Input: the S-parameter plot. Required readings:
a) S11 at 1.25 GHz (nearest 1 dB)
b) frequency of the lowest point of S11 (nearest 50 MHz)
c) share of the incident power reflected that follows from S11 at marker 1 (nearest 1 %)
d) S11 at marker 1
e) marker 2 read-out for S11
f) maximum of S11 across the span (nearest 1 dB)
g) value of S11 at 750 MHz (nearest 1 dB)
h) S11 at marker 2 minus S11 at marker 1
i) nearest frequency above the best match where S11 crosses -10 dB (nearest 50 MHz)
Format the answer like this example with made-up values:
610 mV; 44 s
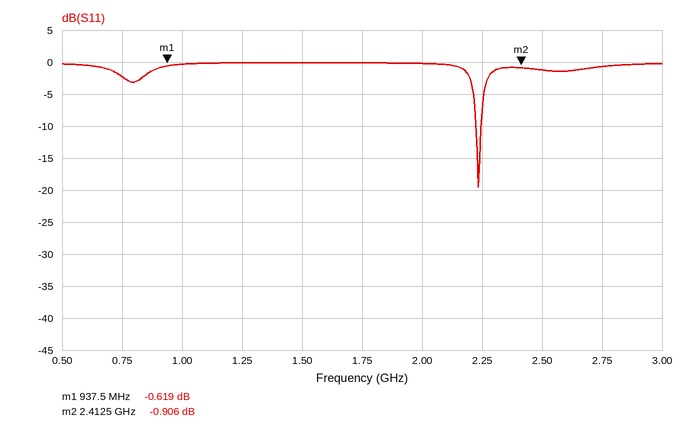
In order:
0 dB; 2.25 GHz; 87 %; -0.619 dB; -0.906 dB; 0 dB; -2 dB; -0.287 dB; 2.25 GHz
